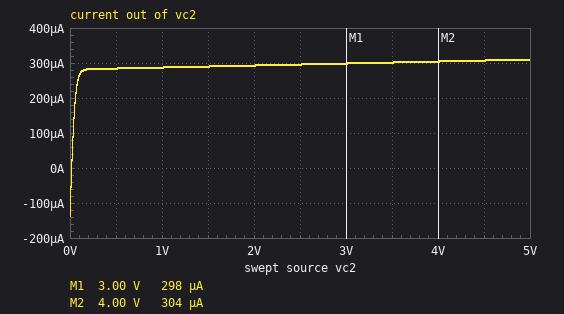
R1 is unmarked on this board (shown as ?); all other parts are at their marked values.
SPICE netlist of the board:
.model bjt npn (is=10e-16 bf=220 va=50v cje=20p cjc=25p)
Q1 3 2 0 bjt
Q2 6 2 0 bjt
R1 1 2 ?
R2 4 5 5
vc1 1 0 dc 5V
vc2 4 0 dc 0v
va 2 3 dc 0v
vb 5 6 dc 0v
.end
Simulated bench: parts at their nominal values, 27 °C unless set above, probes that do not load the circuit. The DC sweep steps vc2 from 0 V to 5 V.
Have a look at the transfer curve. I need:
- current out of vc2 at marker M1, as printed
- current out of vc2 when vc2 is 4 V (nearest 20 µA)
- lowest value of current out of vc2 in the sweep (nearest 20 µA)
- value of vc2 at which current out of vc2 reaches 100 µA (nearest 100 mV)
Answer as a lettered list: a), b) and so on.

a) 298 µA
b) 300 µA
c) -140 µA
d) 0 V
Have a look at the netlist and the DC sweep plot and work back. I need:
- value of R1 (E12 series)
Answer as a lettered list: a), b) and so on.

a) 15 kΩ
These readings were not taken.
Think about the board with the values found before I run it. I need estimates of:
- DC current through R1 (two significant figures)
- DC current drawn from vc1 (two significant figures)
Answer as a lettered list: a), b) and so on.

a) 290 µA
b) 290 µA
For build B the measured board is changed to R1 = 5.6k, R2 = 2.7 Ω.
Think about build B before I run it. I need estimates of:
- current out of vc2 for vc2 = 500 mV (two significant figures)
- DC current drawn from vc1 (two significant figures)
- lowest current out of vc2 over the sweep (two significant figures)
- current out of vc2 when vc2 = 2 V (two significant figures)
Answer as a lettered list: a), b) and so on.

a) 760 µA
b) 770 µA
c) -360 µA
d) 780 µA
